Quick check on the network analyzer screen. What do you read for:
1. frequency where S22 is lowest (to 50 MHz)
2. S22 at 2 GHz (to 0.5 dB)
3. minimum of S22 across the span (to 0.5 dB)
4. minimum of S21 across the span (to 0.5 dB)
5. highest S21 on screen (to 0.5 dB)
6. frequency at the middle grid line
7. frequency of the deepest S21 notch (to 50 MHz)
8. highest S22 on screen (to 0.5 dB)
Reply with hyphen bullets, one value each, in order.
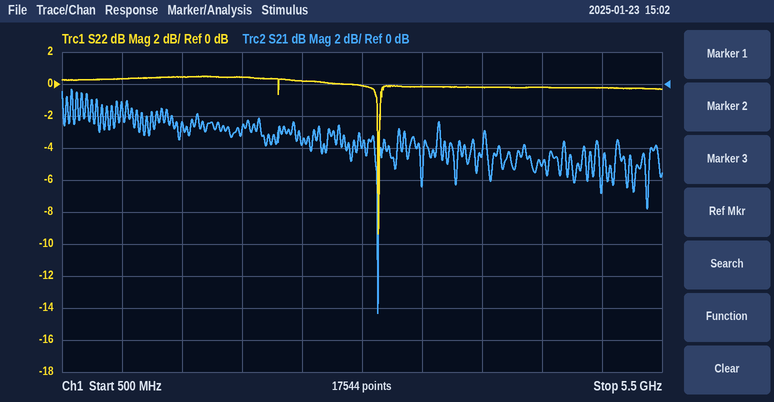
- 3.15 GHz
- 0.5 dB
- -9.5 dB
- -14.5 dB
- -0.5 dB
- 3 GHz
- 3.15 GHz
- 0.5 dB
